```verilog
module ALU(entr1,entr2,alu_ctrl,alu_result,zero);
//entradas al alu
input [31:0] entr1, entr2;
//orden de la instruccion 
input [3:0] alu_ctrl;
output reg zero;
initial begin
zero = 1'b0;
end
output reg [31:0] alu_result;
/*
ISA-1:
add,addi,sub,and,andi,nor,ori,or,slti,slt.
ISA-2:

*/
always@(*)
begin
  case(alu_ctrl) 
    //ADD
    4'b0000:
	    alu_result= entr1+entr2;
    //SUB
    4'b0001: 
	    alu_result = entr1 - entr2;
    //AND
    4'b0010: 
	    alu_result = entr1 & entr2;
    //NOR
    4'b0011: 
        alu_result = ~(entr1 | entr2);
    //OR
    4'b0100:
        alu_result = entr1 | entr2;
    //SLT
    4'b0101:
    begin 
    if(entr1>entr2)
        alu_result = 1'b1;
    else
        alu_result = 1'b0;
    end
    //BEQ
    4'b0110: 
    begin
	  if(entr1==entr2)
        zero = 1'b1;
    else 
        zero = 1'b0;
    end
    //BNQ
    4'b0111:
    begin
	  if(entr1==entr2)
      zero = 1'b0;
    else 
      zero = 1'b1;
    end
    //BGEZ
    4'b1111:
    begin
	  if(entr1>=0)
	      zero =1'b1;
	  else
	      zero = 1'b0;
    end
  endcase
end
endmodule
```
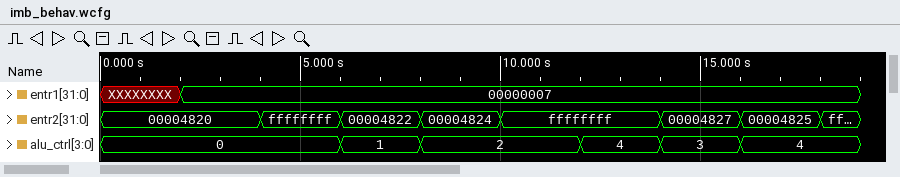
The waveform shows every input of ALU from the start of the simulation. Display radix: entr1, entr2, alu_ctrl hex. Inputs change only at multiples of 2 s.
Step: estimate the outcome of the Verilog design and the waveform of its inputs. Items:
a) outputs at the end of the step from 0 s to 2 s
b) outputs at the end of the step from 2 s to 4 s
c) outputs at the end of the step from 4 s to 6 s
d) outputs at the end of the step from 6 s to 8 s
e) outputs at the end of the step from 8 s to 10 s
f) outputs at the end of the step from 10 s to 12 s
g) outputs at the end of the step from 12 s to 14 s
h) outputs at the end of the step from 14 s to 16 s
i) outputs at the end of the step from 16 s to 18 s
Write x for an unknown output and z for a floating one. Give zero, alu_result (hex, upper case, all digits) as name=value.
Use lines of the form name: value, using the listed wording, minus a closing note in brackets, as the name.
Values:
outputs at the end of the step from 0 s to 2 s: zero=0, alu_result=x
outputs at the end of the step from 2 s to 4 s: zero=0, alu_result=00004827
outputs at the end of the step from 4 s to 6 s: zero=0, alu_result=00000006
outputs at the end of the step from 6 s to 8 s: zero=0, alu_result=FFFFB7E5
outputs at the end of the step from 8 s to 10 s: zero=0, alu_result=00000004
outputs at the end of the step from 10 s to 12 s: zero=0, alu_result=00000007
outputs at the end of the step from 12 s to 14 s: zero=0, alu_result=FFFFFFFF
outputs at the end of the step from 14 s to 16 s: zero=0, alu_result=FFFFB7D8
outputs at the end of the step from 16 s to 18 s: zero=0, alu_result=00004827
